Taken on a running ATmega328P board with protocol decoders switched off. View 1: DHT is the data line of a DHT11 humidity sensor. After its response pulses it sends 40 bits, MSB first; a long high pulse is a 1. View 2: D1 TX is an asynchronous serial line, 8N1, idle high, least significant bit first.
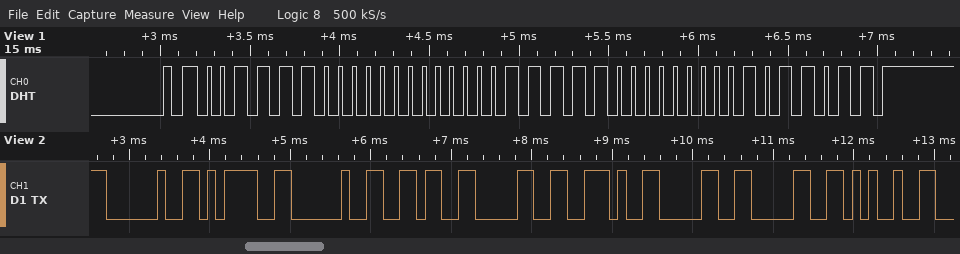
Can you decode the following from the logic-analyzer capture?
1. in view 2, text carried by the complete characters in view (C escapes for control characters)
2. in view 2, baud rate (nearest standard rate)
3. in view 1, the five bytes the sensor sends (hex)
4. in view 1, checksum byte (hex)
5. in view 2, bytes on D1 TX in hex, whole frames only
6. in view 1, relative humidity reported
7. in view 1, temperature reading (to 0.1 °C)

" = 60.00%"
9600 baud
3C 00 1F 00 5B
0x5B
0x20 0x3D 0x20 0x36 0x30 0x2E 0x30 0x30 0x25
60 %
31.0 °C
